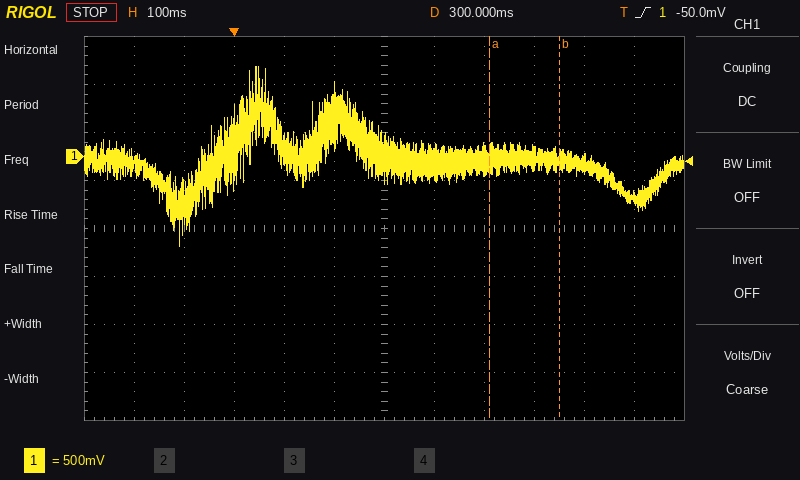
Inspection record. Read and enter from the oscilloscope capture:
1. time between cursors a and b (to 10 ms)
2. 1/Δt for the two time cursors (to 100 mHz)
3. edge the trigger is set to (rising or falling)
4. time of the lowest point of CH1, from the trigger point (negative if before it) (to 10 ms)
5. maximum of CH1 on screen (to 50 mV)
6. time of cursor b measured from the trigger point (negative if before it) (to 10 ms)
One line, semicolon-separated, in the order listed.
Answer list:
140 ms; 7.1 Hz; rising; -110 ms; 950 mV; +650 ms
